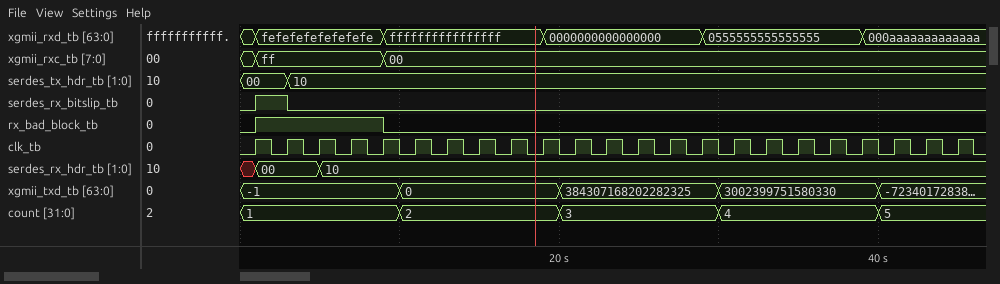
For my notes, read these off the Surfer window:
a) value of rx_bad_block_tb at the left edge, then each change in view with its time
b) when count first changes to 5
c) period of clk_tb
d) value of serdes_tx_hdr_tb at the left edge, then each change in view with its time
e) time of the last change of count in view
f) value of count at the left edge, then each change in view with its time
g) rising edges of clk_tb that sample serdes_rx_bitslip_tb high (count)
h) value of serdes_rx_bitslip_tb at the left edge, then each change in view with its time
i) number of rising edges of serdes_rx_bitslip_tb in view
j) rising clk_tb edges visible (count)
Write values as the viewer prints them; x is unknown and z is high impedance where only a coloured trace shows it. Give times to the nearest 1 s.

0, 1 at 1 s, 0 at 9 s
40 s
2 s
00, 10 at 3 s
40 s
1, 2 at 10 s, 3 at 20 s, 4 at 30 s, 5 at 40 s
1
0, 1 at 1 s, 0 at 3 s
1
23
